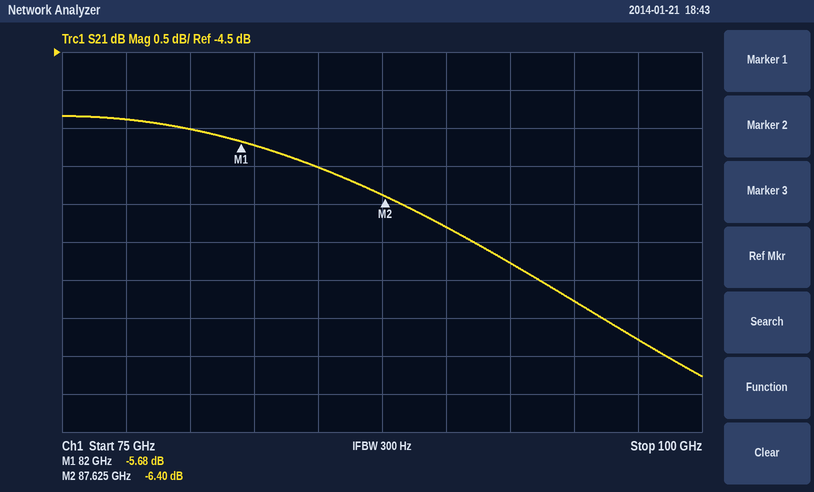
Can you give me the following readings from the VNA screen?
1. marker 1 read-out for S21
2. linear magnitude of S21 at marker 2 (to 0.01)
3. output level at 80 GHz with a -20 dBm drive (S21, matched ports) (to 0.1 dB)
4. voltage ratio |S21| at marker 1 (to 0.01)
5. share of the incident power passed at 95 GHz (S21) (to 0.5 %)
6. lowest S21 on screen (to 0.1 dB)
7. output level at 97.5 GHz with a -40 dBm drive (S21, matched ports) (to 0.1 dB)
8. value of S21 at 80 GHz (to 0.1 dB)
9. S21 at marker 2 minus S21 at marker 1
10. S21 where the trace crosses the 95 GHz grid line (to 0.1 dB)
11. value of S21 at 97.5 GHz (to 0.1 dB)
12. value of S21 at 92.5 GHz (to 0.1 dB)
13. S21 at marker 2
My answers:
-5.68 dB
0.48
-25.5 dBm
0.52
16.5 %
-8.8 dB
-48.3 dBm
-5.5 dB
-0.72 dB
-7.8 dB
-8.3 dB
-7.3 dB
-6.40 dB
